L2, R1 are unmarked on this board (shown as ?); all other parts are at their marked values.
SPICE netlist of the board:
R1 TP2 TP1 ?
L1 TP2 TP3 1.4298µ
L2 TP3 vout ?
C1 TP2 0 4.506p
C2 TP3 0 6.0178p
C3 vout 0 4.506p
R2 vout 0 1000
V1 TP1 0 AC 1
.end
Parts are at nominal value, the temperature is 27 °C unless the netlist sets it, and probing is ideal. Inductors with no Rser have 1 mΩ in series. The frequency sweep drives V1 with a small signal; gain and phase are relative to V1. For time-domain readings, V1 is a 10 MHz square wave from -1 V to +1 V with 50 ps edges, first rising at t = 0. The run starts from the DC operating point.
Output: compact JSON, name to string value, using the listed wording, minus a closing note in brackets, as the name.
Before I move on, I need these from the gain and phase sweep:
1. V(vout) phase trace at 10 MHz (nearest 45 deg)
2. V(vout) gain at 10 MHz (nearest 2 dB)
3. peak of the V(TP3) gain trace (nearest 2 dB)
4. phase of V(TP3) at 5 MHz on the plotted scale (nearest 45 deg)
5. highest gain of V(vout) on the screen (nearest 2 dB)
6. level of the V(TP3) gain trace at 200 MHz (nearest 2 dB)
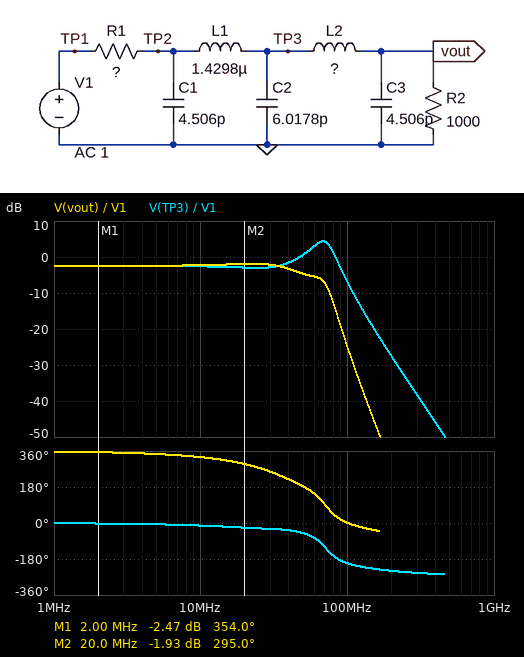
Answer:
{"V(vout) phase trace at 10 MHz": "315 deg", "V(vout) gain at 10 MHz": "-2 dB", "peak of the V(TP3) gain trace": "4 dB", "phase of V(TP3) at 5 MHz on the plotted scale": "0 deg", "highest gain of V(vout) on the screen": "-2 dB", "level of the V(TP3) gain trace at 200 MHz": "-28 dB"}
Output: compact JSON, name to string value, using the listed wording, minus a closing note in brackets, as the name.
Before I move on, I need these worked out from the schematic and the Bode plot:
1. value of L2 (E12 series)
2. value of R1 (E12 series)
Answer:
{"value of L2": "4.7 µH", "value of R1": "330 Ω"}
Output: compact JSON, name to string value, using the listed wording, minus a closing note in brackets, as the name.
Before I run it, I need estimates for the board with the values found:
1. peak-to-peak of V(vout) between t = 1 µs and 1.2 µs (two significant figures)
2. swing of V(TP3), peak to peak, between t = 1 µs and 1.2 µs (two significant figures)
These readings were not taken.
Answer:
{"peak-to-peak of V(vout) between t = 1 µs and 1.2 µs": "1.9 V", "swing of V(TP3), peak to peak, between t = 1 µs and 1.2 µs": "2.5 V"}
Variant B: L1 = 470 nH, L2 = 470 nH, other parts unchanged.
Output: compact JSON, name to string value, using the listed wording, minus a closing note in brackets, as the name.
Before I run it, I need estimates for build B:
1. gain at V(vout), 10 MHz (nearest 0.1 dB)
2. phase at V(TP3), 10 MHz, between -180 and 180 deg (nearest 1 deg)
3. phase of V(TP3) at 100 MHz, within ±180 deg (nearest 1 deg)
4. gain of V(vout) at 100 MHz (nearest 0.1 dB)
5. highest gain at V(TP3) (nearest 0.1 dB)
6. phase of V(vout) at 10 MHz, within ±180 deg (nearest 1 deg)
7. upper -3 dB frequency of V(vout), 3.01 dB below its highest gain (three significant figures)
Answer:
{"gain at V(vout), 10 MHz": "-2.6 dB", "phase at V(TP3), 10 MHz, between -180 and 180 deg": "-14 deg", "phase of V(TP3) at 100 MHz, within ±180 deg": "-91 deg", "gain of V(vout) at 100 MHz": "-2.2 dB", "highest gain at V(TP3)": "1.5 dB", "phase of V(vout) at 10 MHz, within ±180 deg": "-16 deg", "upper -3 dB frequency of V(vout), 3.01 dB below its highest gain": "175 MHz"}
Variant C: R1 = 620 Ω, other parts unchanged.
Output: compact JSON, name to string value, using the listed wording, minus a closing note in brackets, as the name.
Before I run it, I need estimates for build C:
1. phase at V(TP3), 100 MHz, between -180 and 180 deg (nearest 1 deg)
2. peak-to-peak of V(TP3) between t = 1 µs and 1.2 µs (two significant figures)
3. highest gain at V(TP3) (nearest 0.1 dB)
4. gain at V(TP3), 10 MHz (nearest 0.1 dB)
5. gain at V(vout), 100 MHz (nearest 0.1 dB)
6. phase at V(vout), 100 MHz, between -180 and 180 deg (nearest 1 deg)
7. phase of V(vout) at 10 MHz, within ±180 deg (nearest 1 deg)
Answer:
{"phase at V(TP3), 100 MHz, between -180 and 180 deg": "144 deg", "peak-to-peak of V(TP3) between t = 1 µs and 1.2 µs": "1.7 V", "highest gain at V(TP3)": "0.7 dB", "gain at V(TP3), 10 MHz": "-4.6 dB", "gain at V(vout), 100 MHz": "-26.1 dB", "phase at V(vout), 100 MHz, between -180 and 180 deg": "-14 deg", "phase of V(vout) at 10 MHz, within ±180 deg": "-34 deg"}
